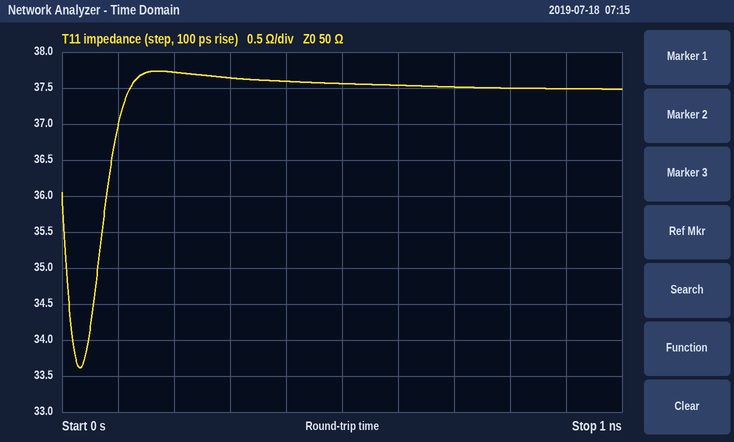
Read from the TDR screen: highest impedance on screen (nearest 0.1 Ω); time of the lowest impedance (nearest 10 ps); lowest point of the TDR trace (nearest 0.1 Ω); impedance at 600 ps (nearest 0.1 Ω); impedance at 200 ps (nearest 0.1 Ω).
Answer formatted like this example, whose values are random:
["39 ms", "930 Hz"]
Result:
["37.7 Ω", "30 ps", "33.6 Ω", "37.5 Ω", "37.7 Ω"]
